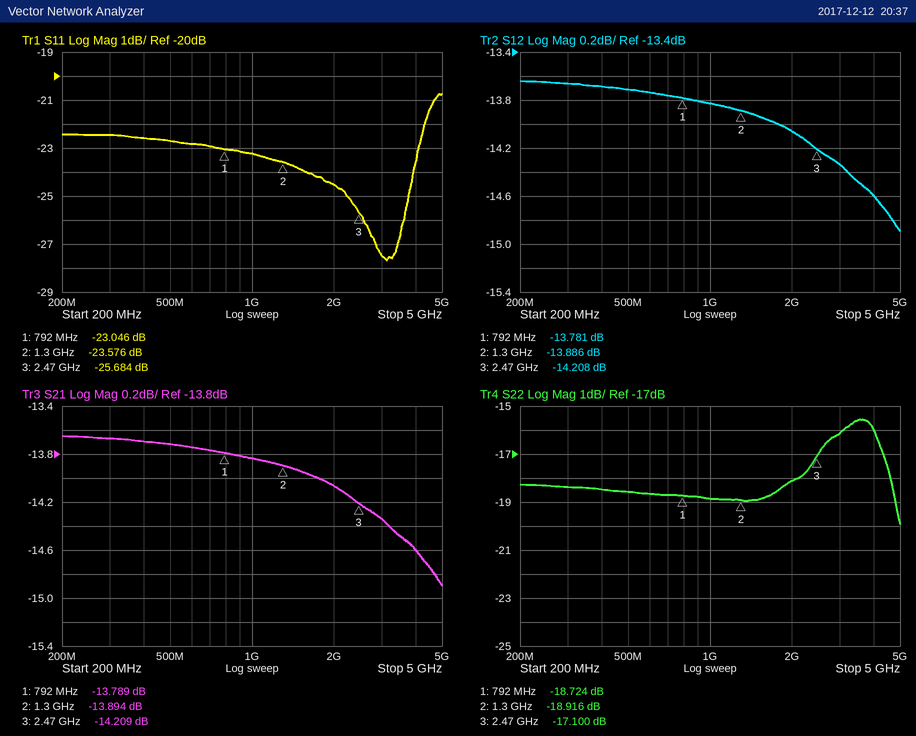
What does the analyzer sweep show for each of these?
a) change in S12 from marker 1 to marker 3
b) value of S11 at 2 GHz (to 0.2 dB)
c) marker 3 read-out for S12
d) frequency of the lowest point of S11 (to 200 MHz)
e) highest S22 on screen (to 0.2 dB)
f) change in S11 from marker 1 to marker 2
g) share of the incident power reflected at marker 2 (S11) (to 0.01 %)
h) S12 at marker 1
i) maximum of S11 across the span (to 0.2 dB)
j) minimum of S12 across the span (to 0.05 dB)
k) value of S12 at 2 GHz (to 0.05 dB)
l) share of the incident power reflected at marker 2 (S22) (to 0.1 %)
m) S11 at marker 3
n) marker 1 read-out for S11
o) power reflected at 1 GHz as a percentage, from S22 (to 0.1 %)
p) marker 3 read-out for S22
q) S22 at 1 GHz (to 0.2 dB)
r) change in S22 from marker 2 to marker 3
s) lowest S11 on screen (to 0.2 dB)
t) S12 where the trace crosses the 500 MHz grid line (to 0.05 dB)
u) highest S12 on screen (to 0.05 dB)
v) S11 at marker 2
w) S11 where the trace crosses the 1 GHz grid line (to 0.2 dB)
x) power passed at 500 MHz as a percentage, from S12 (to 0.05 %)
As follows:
-0.427 dB
-24.6 dB
-14.208 dB
3.2 GHz
-15.6 dB
-0.530 dB
0.44 %
-13.781 dB
-20.8 dB
-14.90 dB
-14.05 dB
1.3 %
-25.684 dB
-23.046 dB
1.3 %
-17.100 dB
-18.8 dB
1.816 dB
-27.6 dB
-13.70 dB
-13.65 dB
-23.576 dB
-23.2 dB
4.25 %
